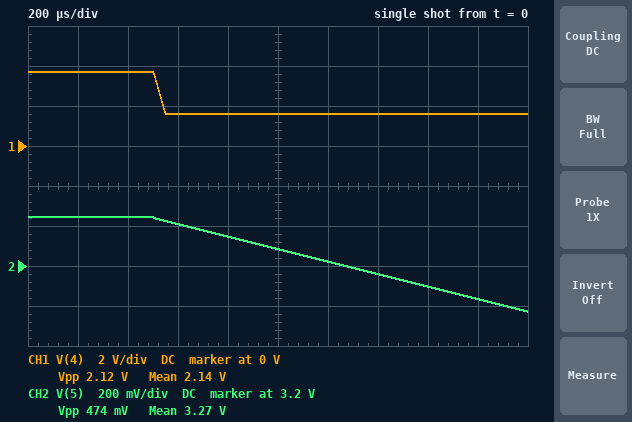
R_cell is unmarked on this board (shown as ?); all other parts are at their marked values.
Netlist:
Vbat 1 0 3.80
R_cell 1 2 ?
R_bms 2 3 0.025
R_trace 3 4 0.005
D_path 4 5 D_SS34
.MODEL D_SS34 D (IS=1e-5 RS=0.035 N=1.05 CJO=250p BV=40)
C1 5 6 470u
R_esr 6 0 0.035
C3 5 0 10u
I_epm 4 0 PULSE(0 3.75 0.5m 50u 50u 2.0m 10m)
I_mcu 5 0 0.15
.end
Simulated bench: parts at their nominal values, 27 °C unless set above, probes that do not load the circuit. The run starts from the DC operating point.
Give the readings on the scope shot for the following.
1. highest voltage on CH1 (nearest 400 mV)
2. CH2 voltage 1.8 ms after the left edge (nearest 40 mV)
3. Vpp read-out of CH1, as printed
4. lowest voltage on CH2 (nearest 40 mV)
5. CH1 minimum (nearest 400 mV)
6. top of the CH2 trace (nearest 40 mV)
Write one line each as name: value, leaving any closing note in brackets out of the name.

highest voltage on CH1: 3.6 V
CH2 voltage 1.8 ms after the left edge: 3.04 V
Vpp read-out of CH1, as printed: 2.12 V
lowest voltage on CH2: 2.96 V
CH1 minimum: 1.6 V
top of the CH2 trace: 3.44 V
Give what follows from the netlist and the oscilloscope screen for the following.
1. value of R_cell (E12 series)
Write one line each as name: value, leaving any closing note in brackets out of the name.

value of R_cell: 0.56 Ω
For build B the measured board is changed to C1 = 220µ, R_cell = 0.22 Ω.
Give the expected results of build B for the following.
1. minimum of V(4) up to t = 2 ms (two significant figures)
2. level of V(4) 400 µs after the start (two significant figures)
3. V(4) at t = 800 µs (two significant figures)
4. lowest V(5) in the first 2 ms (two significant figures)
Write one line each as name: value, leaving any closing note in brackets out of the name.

minimum of V(4) up to t = 2 ms: 2.8 V
level of V(4) 400 µs after the start: 3.8 V
V(4) at t = 800 µs: 2.9 V
lowest V(5) in the first 2 ms: 2.6 V
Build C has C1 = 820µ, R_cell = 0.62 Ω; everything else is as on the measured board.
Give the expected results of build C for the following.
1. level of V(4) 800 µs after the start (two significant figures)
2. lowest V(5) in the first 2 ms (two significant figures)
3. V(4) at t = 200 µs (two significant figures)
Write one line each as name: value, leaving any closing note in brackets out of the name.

level of V(4) 800 µs after the start: 1.4 V
lowest V(5) in the first 2 ms: 3.2 V
V(4) at t = 200 µs: 3.7 V
